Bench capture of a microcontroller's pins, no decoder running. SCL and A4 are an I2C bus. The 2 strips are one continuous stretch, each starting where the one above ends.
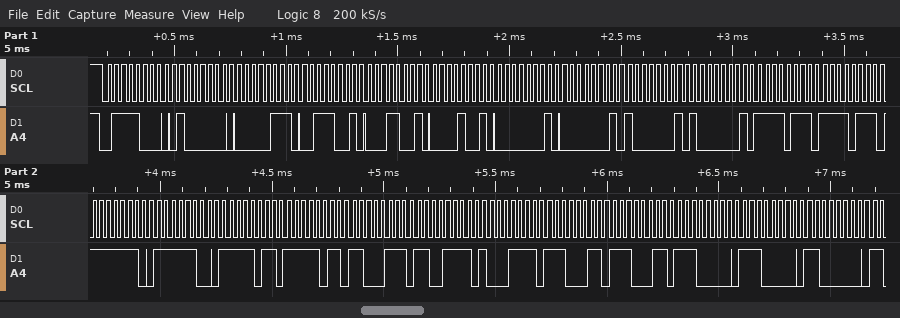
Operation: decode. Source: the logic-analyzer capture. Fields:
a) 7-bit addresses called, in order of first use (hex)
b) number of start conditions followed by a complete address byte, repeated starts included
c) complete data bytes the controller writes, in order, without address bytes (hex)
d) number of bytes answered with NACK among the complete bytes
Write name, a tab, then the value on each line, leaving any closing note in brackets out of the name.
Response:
7-bit addresses called, in order of first use	0x3C
number of start conditions followed by a complete address byte, repeated starts included	1
complete data bytes the controller writes, in order, without address bytes	40 07 39 19 09 01 01 81 81 F7 F7 FE FC FB FB C7 CF 8F E3 E3 E0 E0 C0
number of bytes answered with NACK among the complete bytes	0
